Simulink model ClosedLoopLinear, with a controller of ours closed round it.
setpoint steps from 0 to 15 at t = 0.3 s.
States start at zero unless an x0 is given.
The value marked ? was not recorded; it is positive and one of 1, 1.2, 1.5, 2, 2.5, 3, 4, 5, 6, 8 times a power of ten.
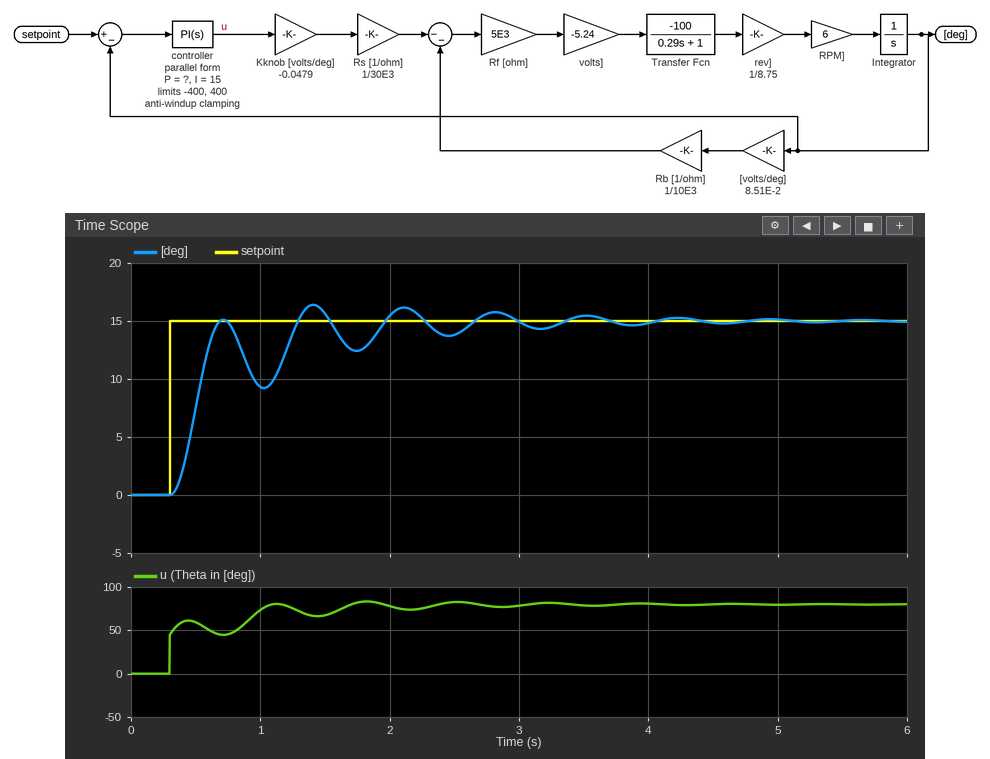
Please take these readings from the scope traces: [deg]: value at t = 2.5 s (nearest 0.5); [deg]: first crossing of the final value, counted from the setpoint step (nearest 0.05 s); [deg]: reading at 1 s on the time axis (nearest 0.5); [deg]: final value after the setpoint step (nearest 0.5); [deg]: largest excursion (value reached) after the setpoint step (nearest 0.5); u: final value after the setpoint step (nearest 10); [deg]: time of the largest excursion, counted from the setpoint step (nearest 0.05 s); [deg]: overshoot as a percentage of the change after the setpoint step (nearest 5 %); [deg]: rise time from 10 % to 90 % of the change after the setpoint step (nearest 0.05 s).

14.0
0.40 s
9.5
15.0
16.5
80
1.10 s
10 %
0.25 s
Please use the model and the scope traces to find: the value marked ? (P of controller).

3
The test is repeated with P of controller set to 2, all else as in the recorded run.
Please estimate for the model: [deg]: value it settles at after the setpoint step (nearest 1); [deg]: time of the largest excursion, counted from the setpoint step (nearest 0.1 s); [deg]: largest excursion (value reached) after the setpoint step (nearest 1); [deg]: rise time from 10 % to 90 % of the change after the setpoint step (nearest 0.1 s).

15
1.2 s
17
0.3 s
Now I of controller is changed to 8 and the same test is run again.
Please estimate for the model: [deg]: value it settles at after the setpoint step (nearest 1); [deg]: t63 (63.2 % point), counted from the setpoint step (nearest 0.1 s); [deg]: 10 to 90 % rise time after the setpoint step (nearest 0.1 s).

15
0.3 s
1.6 s
